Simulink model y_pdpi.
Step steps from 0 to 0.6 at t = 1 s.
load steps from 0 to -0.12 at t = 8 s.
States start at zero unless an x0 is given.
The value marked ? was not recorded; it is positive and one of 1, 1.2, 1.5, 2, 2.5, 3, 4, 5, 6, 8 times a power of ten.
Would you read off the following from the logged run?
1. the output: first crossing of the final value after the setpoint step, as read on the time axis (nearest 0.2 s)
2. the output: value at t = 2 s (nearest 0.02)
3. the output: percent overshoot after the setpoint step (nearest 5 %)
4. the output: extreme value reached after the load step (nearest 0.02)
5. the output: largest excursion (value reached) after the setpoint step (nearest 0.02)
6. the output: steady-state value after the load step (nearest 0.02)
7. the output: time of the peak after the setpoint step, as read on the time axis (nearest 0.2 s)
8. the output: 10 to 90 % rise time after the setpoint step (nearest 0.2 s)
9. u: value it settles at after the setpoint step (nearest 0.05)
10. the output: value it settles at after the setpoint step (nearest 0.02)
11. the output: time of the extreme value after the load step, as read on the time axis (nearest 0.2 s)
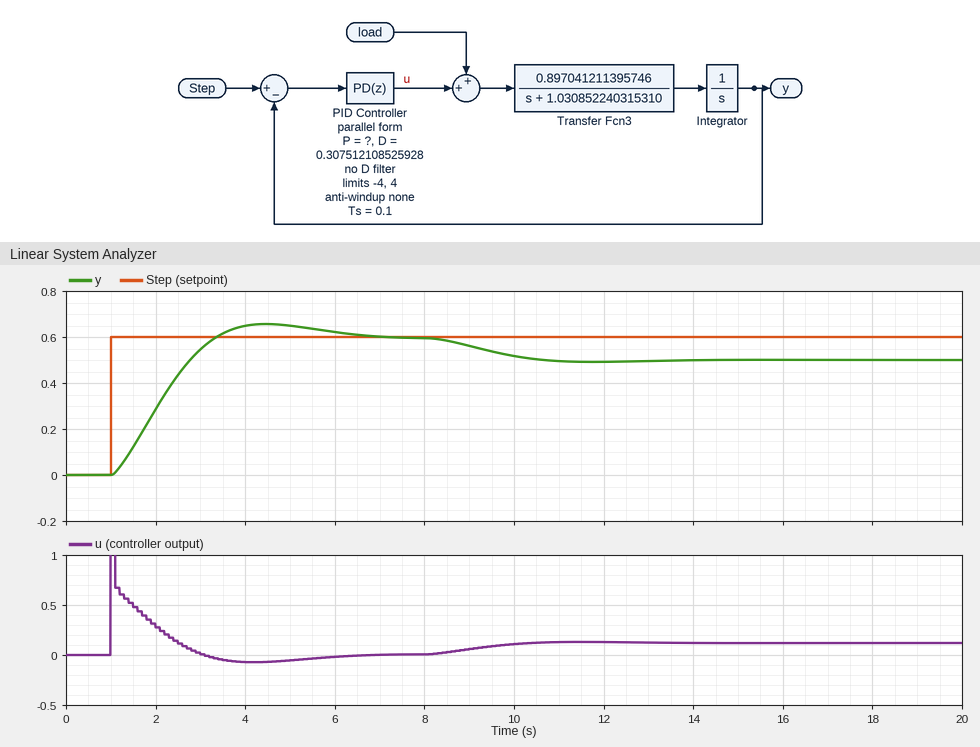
3.4 s
0.28
10 %
0.50
0.66
0.50
4.4 s
1.6 s
0.00
0.60
11.8 s
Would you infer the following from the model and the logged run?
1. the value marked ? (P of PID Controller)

1.2
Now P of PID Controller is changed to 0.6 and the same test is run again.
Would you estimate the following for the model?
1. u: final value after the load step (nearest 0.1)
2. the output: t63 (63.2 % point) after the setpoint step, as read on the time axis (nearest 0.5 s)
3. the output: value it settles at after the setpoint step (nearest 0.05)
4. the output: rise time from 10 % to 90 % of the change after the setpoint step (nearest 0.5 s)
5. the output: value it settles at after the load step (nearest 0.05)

0.1
3.0 s
0.60
3.5 s
0.40
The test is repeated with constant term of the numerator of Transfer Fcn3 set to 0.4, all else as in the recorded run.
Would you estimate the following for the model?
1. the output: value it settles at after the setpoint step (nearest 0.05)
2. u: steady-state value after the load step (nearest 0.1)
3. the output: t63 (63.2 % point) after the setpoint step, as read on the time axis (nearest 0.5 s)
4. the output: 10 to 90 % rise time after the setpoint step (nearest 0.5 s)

0.60
0.1
3.5 s
3.5 s
